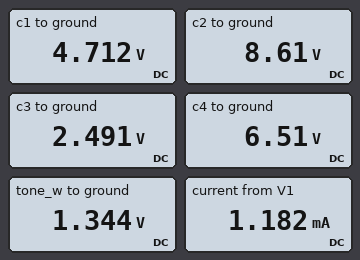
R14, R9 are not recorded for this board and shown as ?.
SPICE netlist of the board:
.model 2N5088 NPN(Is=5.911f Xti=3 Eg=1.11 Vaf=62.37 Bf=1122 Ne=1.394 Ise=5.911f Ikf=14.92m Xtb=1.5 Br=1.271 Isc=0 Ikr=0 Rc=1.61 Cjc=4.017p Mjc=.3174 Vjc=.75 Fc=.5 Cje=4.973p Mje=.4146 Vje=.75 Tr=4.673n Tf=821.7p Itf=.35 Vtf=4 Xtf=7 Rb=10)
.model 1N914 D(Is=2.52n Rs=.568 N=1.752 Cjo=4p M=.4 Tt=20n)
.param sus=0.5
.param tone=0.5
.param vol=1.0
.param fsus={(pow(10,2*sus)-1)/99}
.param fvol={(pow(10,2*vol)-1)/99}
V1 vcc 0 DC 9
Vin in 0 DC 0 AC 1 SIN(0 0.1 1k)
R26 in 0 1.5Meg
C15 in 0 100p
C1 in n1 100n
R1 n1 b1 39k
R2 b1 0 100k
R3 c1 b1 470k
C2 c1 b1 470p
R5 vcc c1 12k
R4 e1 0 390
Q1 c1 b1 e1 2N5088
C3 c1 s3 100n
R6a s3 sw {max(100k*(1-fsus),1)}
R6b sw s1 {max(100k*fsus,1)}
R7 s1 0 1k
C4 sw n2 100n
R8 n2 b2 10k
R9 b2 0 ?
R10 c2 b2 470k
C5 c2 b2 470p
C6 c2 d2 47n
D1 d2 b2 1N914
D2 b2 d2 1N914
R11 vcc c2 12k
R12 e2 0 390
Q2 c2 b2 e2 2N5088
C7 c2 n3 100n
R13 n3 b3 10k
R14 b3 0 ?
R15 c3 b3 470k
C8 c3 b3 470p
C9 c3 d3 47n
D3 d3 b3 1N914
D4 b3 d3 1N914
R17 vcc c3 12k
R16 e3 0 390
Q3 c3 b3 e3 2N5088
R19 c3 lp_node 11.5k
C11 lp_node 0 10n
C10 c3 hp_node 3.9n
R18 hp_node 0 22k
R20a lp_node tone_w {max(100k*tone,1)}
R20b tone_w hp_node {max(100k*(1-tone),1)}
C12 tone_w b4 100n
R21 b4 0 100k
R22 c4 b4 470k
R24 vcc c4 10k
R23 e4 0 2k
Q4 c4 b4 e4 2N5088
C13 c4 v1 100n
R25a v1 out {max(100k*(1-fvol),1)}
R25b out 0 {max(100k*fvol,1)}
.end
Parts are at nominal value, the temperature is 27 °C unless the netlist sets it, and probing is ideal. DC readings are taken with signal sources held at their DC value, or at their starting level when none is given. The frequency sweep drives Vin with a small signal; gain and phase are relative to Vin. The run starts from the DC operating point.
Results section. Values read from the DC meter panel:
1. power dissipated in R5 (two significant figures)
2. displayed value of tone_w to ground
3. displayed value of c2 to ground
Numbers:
1.5 mW
1.344 V
8.61 V
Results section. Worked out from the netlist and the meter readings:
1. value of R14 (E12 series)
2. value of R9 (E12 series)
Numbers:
330 kΩ
33 kΩ
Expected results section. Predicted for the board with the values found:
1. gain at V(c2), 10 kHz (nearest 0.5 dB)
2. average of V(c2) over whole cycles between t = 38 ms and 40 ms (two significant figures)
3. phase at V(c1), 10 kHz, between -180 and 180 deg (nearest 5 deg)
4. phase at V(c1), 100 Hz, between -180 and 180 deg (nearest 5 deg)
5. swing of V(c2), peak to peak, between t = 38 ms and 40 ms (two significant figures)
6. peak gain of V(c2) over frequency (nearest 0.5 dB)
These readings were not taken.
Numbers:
-23.0 dB
8.6 V
95 deg
-170 deg
160 mV
2.5 dB
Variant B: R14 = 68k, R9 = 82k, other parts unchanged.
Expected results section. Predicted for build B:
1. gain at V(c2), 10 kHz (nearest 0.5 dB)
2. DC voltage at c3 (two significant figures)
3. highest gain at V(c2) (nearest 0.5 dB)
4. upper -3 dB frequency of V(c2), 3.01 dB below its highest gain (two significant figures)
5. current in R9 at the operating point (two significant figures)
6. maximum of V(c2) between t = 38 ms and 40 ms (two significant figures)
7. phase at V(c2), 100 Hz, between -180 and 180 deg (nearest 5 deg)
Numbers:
-18.5 dB
5.8 V
14.0 dB
990 Hz
9.2 µA
5.5 V
35 deg
